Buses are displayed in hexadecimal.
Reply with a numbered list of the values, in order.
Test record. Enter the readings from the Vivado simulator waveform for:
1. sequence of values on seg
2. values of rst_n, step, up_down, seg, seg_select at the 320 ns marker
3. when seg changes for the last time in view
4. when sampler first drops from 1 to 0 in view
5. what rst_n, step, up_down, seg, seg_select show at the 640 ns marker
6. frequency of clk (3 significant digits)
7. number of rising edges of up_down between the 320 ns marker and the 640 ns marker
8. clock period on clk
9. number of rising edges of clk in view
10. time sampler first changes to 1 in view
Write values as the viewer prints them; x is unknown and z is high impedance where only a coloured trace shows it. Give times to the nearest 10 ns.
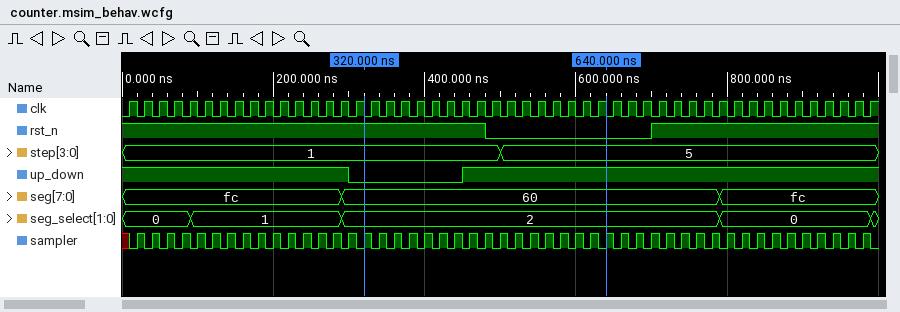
1. fc, 60, fc
2. rst_n=1, step=1, up_down=0, seg=60, seg_select=2
3. 790 ns
4. 30 ns
5. rst_n=0, step=5, up_down=1, seg=60, seg_select=2
6. 50.0 MHz
7. 1
8. 20 ns
9. 50
10. 20 ns
